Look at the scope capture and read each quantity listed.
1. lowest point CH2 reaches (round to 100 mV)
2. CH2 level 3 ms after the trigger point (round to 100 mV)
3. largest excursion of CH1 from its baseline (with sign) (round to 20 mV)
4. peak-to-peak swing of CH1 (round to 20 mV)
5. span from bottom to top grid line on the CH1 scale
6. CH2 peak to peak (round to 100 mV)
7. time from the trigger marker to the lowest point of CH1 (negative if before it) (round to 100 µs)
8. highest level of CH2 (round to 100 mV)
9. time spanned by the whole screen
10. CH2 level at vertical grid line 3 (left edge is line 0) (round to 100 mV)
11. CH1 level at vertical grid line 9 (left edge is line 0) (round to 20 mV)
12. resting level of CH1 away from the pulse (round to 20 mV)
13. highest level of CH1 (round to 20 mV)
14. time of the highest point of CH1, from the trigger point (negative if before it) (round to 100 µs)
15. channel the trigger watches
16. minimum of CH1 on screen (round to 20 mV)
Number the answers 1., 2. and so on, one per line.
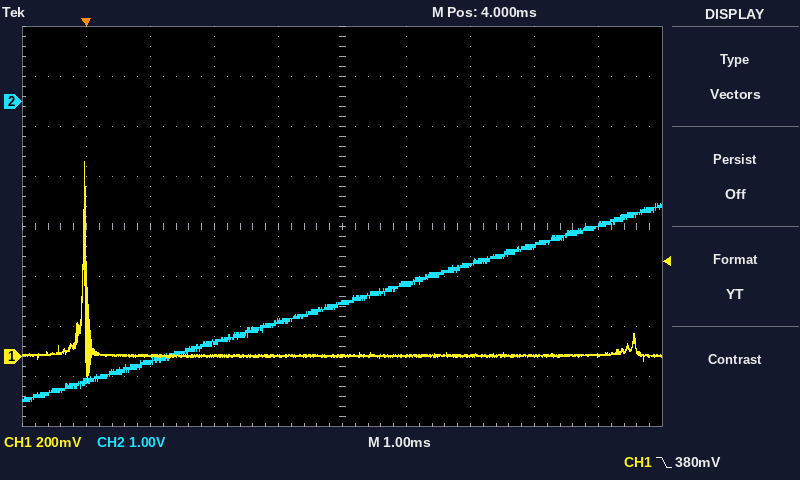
1. -6.0 V
2. -4.4 V
3. +780 mV
4. 880 mV
5. 1.6 V
6. 4.0 V
7. 0.0 ms
8. -2.0 V
9. 10 ms
10. -4.8 V
11. 0 mV
12. 0 mV
13. 780 mV
14. 0.0 ms
15. CH1
16. -100 mV
